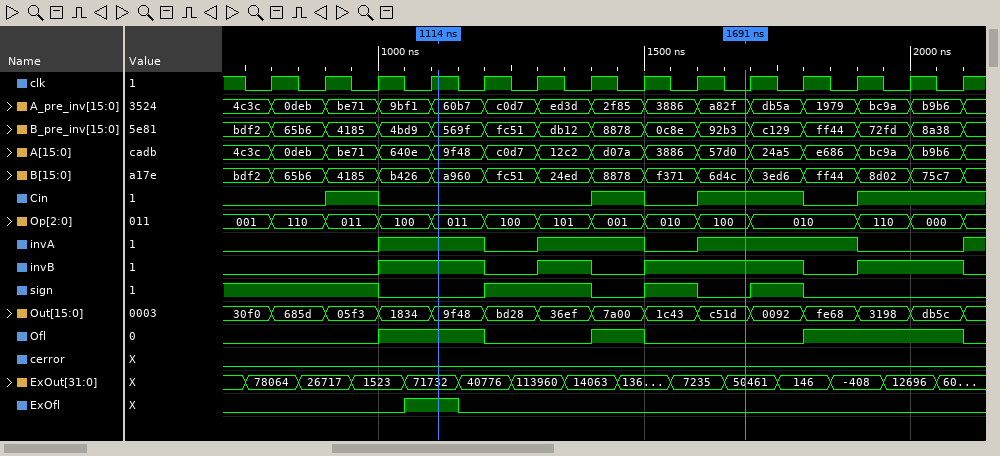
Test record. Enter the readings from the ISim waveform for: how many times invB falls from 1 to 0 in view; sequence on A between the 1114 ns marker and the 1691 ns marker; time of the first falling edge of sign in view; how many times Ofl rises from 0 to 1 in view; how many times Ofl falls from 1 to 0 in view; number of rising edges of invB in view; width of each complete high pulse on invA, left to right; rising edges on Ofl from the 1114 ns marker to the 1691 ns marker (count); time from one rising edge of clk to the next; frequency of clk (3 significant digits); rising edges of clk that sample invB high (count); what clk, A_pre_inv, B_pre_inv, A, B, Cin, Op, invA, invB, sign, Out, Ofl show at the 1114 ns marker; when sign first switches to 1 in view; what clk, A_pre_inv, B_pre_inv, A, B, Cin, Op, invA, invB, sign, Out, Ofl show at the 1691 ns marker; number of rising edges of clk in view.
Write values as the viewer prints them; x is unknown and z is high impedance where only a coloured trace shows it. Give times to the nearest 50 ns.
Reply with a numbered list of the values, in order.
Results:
1. 4
2. 9f48, c0d7, 12c2, d07a, 3886, 57d0
3. 1000 ns
4. 3
5. 3
6. 4
7. 200 ns, 200 ns, 300 ns
8. 1
9. 100 ns
10. 10.0 MHz
11. 8
12. clk=1, A_pre_inv=60b7, B_pre_inv=569f, A=9f48, B=a960, Cin=0, Op=011, invA=1, invB=1, sign=0, Out=9f48, Ofl=1
13. 1200 ns
14. clk=0, A_pre_inv=a82f, B_pre_inv=92b3, A=57d0, B=6d4c, Cin=1, Op=100, invA=1, invB=1, sign=0, Out=c51d, Ofl=0
15. 14
